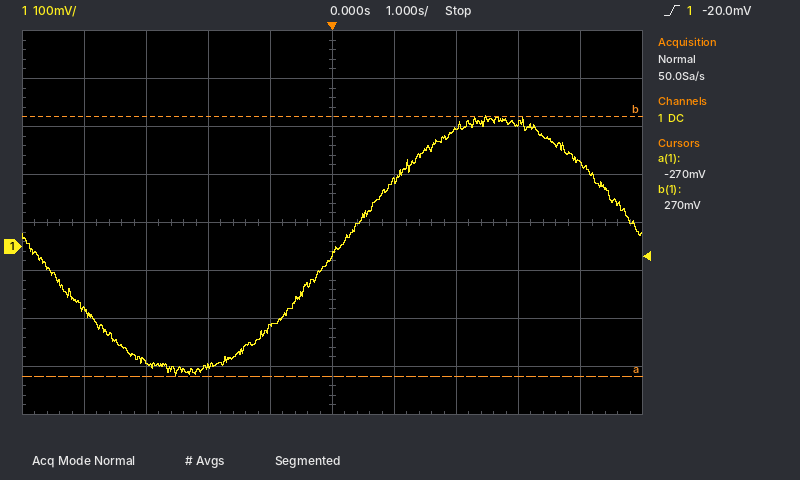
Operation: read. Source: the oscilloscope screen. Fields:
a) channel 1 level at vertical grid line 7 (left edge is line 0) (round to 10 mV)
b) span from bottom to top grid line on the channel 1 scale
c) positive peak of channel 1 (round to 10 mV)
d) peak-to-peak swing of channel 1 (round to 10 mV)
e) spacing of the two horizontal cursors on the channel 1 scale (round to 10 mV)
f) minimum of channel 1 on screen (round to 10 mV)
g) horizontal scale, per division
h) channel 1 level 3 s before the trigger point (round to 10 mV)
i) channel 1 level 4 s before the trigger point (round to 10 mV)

250 mV
800 mV
270 mV
540 mV
540 mV
-270 mV
1 s
-240 mV
-130 mV
